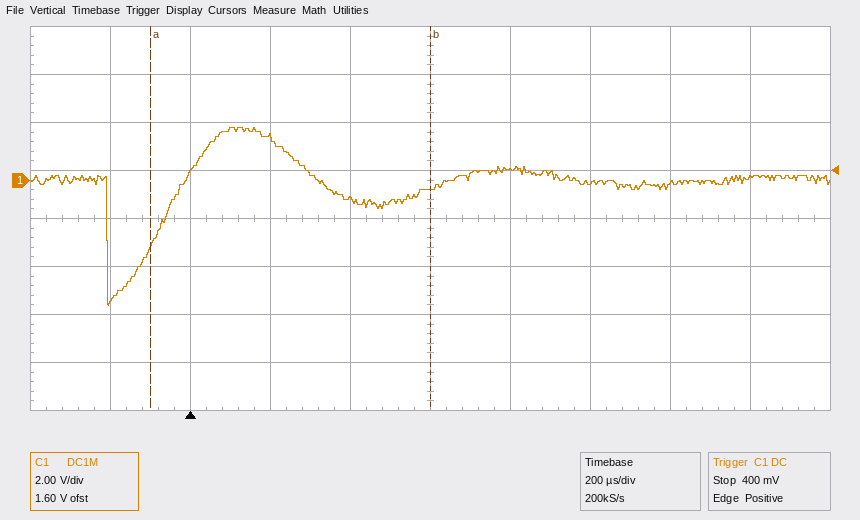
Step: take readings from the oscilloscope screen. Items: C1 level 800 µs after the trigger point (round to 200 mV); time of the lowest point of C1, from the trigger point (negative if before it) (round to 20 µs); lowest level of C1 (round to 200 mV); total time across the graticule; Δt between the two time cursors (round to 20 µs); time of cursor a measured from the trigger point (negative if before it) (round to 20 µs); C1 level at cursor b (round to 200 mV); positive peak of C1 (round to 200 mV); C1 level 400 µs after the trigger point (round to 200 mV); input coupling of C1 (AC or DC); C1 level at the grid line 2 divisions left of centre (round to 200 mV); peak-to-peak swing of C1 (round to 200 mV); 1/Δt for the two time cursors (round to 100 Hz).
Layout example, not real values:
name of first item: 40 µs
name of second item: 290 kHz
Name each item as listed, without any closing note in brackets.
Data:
C1 level 800 µs after the trigger point: 400 mV
time of the lowest point of C1, from the trigger point (negative if before it): -200 µs
lowest level of C1: -5.2 V
total time across the graticule: 2 ms
Δt between the two time cursors: 700 µs
time of cursor a measured from the trigger point (negative if before it): -100 µs
C1 level at cursor b: -400 mV
positive peak of C1: 2.2 V
C1 level 400 µs after the trigger point: -800 mV
input coupling of C1: DC
C1 level at the grid line 2 divisions left of centre: 1.8 V
peak-to-peak swing of C1: 7.4 V
1/Δt for the two time cursors: 1.4 kHz
